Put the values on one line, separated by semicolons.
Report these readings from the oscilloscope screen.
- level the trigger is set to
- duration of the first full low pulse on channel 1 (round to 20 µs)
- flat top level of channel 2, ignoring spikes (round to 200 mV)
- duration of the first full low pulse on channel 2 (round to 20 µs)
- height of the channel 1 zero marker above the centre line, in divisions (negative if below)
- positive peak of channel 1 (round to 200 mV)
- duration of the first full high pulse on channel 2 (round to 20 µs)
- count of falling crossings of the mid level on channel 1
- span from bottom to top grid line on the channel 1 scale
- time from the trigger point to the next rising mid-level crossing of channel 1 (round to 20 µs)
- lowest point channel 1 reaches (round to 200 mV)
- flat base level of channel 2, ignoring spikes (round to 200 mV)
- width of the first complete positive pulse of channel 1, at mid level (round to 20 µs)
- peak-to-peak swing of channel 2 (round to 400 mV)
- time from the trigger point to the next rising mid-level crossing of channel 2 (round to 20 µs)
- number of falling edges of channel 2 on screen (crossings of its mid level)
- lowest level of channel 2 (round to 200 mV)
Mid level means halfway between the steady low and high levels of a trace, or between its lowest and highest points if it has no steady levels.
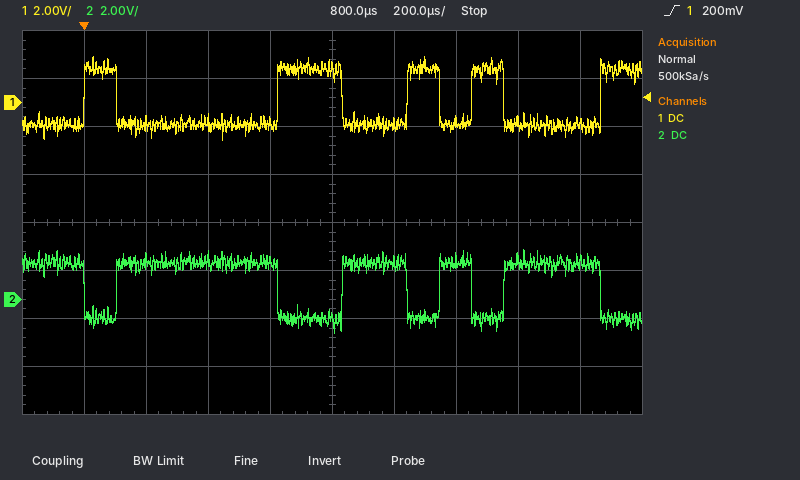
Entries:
200 mV; 520 µs; 1.6 V; 100 µs; +2.5 div; 2.0 V; 520 µs; 4; 16 V; 620 µs; -1.6 V; -800 mV; 100 µs; 3.6 V; 100 µs; 5; -1.4 V
